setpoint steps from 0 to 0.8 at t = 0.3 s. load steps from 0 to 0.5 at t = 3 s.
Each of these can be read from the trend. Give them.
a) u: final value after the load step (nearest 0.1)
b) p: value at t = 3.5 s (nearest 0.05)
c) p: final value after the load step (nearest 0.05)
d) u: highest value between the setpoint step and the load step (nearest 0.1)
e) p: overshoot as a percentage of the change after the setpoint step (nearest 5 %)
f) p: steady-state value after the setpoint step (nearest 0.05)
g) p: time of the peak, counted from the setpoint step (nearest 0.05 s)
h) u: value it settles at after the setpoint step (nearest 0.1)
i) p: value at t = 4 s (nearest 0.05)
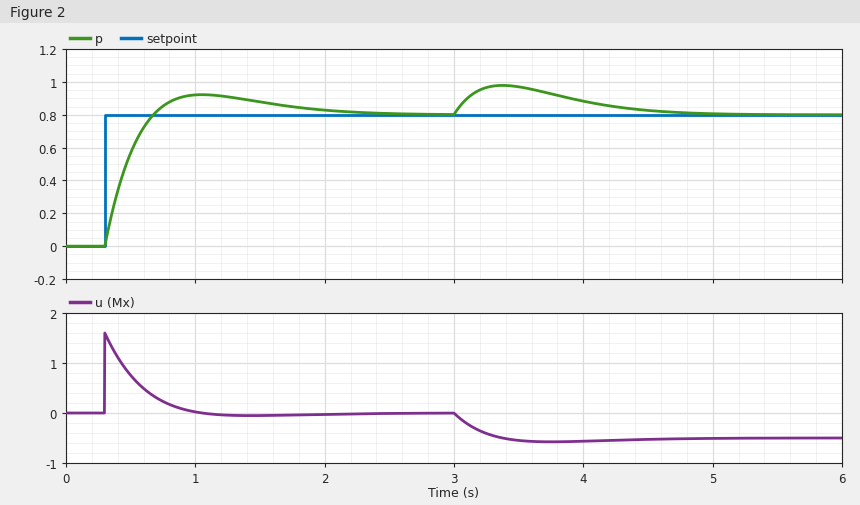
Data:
-0.5
0.95
0.80
1.6
15 %
0.80
0.75 s
0.0
0.90
